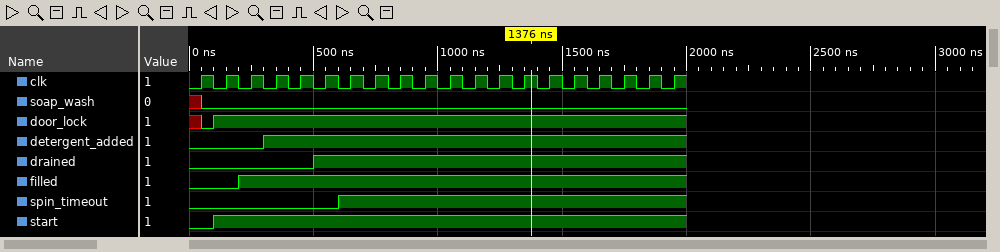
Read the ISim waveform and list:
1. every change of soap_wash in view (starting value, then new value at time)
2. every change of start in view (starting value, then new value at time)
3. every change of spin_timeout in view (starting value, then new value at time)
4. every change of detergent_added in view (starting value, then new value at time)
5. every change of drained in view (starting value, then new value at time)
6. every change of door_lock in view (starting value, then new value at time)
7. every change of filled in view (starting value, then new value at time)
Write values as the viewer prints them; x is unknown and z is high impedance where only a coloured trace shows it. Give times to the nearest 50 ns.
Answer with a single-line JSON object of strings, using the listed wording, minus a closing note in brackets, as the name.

{"every change of soap_wash in view": "x, 0 at 50 ns", "every change of start in view": "0, 1 at 100 ns", "every change of spin_timeout in view": "0, 1 at 600 ns", "every change of detergent_added in view": "0, 1 at 300 ns", "every change of drained in view": "0, 1 at 500 ns", "every change of door_lock in view": "x, 0 at 50 ns, 1 at 100 ns", "every change of filled in view": "0, 1 at 200 ns"}
